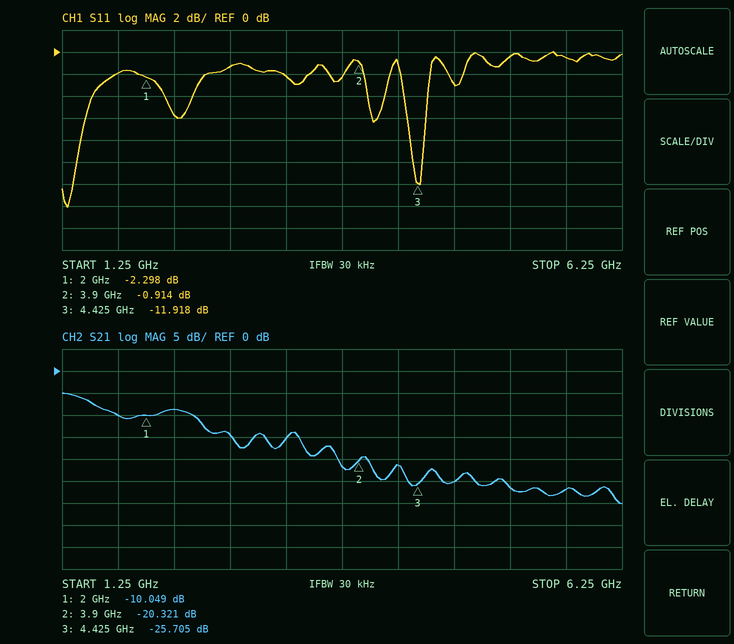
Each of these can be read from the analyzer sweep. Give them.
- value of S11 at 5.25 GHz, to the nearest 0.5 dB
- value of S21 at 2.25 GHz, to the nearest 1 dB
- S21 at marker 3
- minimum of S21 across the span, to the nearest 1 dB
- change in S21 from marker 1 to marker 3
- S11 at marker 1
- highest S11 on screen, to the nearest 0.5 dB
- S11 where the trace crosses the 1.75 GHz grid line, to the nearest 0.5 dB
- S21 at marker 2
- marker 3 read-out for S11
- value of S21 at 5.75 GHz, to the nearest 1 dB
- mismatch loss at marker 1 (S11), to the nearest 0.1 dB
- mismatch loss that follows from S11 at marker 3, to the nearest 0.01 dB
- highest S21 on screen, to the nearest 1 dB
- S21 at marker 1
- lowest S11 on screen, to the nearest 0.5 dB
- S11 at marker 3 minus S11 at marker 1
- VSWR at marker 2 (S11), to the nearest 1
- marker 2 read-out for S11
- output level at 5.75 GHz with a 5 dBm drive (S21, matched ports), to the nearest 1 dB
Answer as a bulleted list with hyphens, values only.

- -0.5 dB
- -9 dB
- -25.705 dB
- -30 dB
- -15.656 dB
- -2.298 dB
- 0.0 dB
- -2.0 dB
- -20.321 dB
- -11.918 dB
- -27 dB
- 3.9 dB
- 0.29 dB
- -5 dB
- -10.049 dB
- -14.0 dB
- -9.620 dB
- 19
- -0.914 dB
- -22 dBm
